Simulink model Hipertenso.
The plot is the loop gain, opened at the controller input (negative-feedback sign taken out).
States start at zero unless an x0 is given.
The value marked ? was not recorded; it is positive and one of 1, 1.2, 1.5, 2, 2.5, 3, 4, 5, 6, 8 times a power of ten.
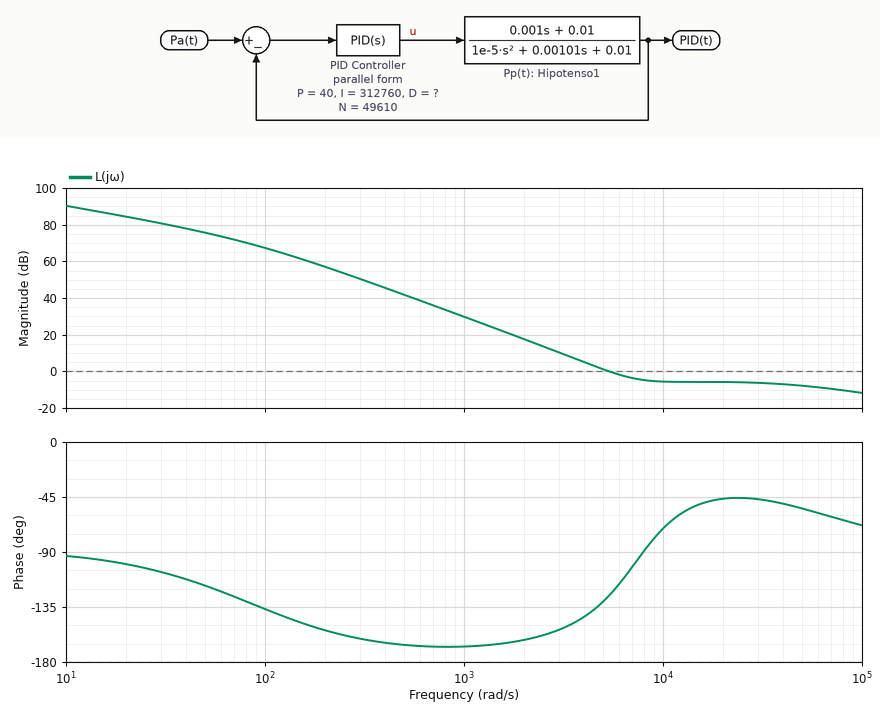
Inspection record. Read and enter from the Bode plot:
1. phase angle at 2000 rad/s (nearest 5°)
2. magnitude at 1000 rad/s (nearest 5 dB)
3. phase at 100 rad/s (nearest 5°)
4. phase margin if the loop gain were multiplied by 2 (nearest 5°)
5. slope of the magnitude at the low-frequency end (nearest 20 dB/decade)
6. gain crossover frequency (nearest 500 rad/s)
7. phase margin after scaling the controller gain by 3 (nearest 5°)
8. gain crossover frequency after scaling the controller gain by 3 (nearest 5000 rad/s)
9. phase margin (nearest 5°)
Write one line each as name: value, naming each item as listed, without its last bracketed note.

phase angle at 2000 rad/s: -160°
magnitude at 1000 rad/s: 30 dB
phase at 100 rad/s: -135°
phase margin if the loop gain were multiplied by 2: 135°
slope of the magnitude at the low-frequency end: -20 dB/decade
gain crossover frequency: 5500 rad/s
phase margin after scaling the controller gain by 3: 120°
gain crossover frequency after scaling the controller gain by 3: 70000 rad/s
phase margin: 55°
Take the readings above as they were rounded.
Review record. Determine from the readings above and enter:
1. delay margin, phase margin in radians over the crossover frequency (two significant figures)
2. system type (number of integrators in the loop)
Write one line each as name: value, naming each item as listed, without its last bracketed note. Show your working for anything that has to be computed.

delay margin, phase margin in radians over the crossover frequency: 55 × π / 180 / 5500 = 0.00017 s
system type: 1
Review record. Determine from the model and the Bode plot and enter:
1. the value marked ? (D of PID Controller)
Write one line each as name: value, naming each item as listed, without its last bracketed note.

the value marked ?: 0.005
